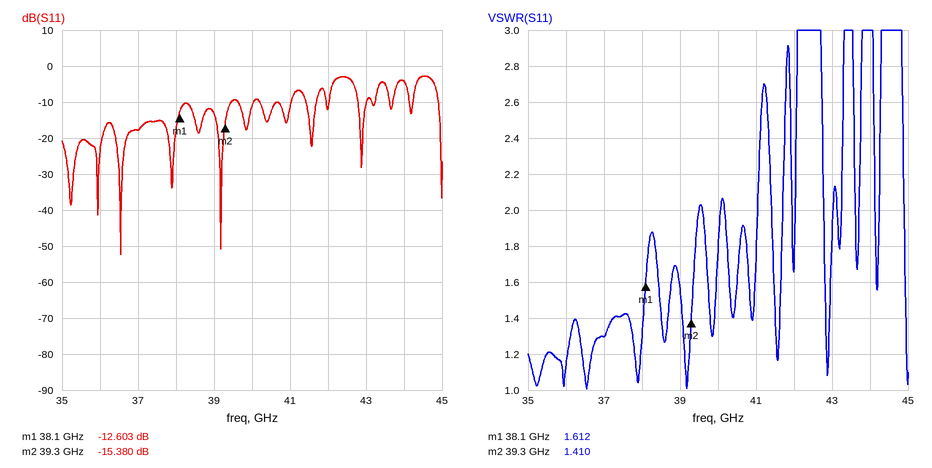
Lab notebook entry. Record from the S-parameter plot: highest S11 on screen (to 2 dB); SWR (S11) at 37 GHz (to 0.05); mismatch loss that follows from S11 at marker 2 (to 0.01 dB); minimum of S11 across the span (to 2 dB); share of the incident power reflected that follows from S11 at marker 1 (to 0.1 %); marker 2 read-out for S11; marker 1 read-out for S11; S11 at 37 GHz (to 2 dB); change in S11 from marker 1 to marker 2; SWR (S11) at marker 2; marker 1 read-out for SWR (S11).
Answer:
-2 dB
1.30
0.13 dB
-52 dB
5.5 %
-15.380 dB
-12.603 dB
-18 dB
-2.777 dB
1.410
1.612
